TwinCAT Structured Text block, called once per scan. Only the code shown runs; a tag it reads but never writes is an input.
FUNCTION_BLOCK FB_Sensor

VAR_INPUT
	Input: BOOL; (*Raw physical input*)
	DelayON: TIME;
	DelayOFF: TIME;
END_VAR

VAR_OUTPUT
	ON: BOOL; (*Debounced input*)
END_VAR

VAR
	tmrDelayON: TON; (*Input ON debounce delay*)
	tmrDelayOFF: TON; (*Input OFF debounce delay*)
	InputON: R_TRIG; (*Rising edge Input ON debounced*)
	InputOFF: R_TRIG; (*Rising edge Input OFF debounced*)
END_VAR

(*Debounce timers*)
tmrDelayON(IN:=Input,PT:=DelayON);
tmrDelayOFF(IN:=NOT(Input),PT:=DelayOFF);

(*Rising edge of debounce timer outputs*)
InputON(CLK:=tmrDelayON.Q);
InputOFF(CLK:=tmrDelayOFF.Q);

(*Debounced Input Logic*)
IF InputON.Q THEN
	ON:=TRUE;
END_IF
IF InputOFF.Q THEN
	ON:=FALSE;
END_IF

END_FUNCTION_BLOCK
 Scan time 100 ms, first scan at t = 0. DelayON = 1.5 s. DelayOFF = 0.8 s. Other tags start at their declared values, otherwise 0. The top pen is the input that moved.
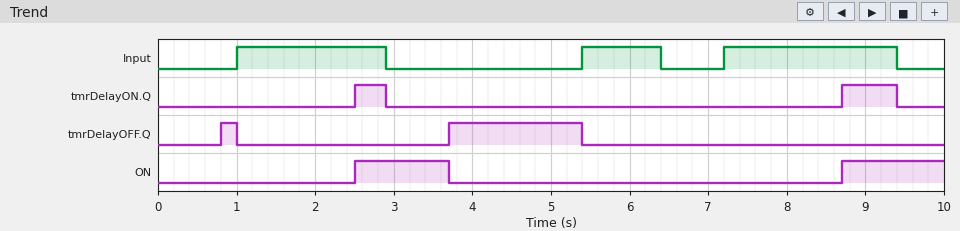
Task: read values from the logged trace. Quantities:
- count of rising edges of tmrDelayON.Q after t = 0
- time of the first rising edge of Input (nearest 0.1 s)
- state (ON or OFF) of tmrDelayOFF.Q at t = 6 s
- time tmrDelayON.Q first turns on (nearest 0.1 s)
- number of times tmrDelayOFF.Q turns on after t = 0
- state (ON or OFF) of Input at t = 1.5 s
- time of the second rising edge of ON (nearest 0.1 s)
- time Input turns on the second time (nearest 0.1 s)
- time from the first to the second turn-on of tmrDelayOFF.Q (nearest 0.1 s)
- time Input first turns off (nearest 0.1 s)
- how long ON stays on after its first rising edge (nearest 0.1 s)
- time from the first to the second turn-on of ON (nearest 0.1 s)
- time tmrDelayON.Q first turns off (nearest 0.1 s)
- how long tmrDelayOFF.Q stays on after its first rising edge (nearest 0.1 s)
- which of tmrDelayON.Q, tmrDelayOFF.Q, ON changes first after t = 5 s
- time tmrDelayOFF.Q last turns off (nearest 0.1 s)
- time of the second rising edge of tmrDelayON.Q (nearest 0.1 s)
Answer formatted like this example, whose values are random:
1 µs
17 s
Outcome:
2
1.0 s
OFF
2.5 s
2
ON
8.7 s
5.4 s
2.9 s
2.9 s
1.2 s
6.2 s
2.9 s
0.2 s
tmrDelayOFF.Q
5.4 s
8.7 s
